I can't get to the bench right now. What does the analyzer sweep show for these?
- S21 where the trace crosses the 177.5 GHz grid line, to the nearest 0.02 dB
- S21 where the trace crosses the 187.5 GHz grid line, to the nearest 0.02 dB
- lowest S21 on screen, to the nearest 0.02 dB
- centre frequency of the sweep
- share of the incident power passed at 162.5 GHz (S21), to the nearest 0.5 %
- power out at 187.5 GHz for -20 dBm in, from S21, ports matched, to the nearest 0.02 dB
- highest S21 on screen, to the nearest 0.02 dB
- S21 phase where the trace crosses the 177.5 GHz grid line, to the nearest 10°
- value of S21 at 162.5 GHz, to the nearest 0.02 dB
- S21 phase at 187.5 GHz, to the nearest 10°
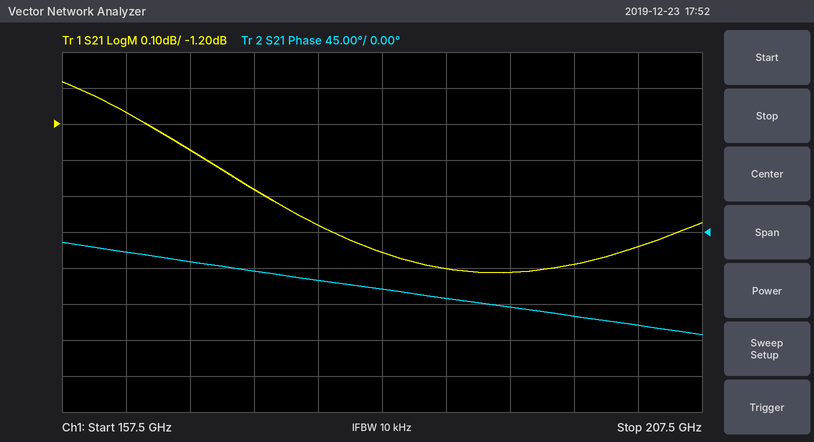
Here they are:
-1.48 dB
-1.60 dB
-1.62 dB
182.5 GHz
76.5 %
-21.60 dBm
-1.08 dB
-60°
-1.16 dB
-80°
